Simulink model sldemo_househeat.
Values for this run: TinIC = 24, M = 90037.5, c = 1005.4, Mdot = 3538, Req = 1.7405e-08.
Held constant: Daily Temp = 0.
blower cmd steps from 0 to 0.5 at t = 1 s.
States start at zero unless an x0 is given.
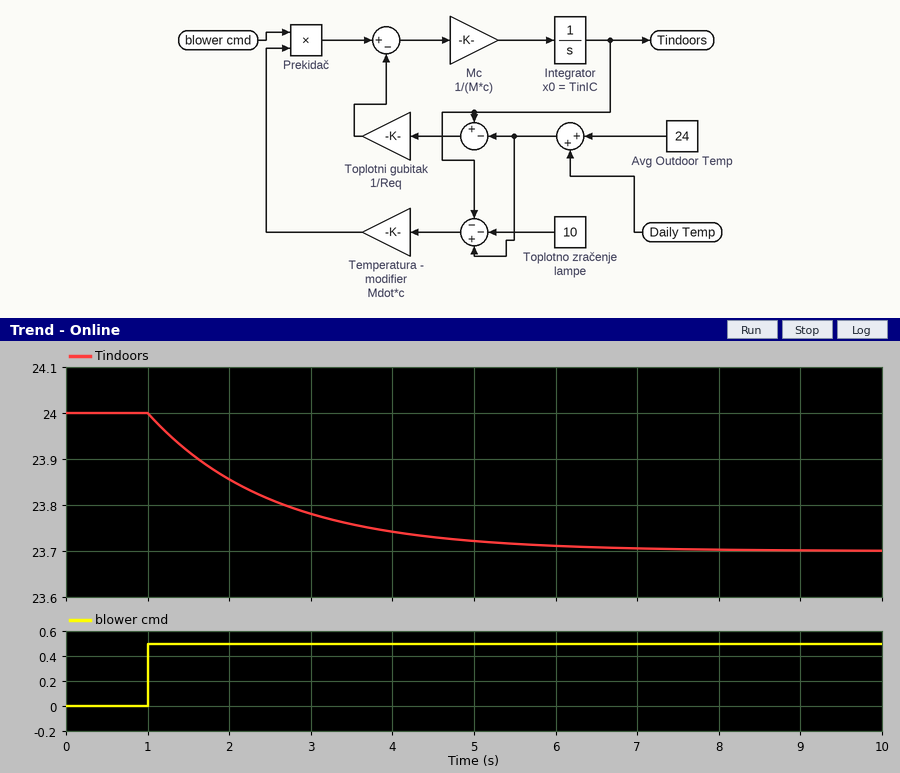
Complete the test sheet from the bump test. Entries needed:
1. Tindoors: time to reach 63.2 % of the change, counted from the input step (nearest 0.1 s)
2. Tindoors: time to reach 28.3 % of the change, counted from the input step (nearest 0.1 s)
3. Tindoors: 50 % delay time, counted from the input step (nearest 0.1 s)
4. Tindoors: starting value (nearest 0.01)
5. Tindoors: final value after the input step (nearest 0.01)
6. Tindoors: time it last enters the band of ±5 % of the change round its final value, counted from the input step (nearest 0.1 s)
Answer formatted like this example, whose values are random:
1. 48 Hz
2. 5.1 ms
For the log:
1. 1.5 s
2. 0.5 s
3. 1.1 s
4. 24.00
5. 23.70
6. 4.6 s
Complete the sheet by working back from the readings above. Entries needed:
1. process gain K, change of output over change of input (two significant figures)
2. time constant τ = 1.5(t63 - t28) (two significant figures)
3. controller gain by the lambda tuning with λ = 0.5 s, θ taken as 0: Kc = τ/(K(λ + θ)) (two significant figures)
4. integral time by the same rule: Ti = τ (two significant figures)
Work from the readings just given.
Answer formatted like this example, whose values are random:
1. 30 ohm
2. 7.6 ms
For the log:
1. -0.60
2. 1.5 s
3. -5.0
4. 1.5 s
